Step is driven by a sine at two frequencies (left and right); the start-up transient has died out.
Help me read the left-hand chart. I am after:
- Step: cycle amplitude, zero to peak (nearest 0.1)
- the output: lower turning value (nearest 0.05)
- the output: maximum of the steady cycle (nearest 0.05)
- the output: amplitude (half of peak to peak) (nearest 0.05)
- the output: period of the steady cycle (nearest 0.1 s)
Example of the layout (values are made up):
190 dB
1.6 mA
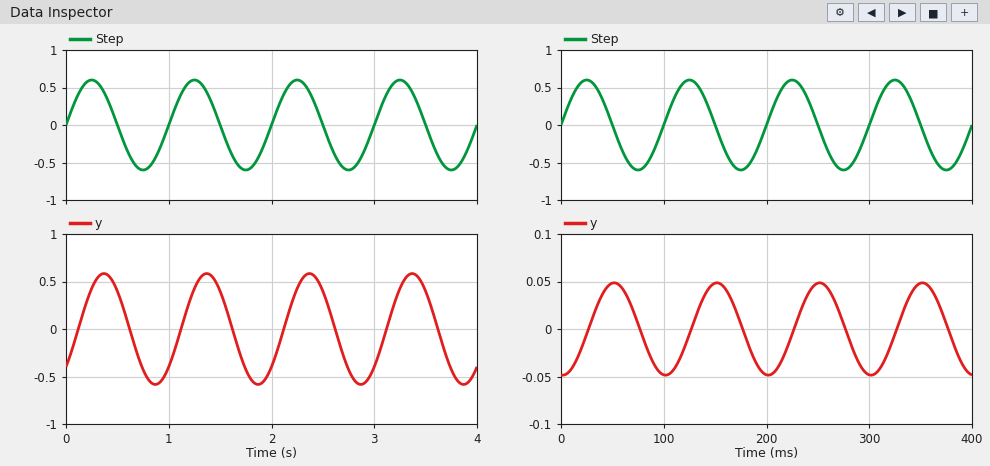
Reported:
0.6
-0.60
0.60
0.60
1.0 s
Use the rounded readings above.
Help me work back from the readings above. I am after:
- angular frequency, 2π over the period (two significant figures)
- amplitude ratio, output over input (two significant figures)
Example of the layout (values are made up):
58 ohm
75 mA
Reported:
6.3 rad/s
1.0
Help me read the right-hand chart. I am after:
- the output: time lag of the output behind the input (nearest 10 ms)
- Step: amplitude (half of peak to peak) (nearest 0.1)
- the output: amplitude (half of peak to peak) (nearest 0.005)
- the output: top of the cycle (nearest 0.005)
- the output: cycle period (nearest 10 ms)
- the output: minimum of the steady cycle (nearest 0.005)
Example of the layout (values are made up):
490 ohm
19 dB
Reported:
30 ms
0.6
0.050
0.050
100 ms
-0.050
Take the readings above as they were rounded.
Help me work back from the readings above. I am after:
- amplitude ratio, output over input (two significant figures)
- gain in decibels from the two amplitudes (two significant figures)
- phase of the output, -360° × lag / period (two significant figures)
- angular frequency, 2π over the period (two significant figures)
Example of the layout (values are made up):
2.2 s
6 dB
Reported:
0.083
-22 dB
-110°
0.063 rad/ms
